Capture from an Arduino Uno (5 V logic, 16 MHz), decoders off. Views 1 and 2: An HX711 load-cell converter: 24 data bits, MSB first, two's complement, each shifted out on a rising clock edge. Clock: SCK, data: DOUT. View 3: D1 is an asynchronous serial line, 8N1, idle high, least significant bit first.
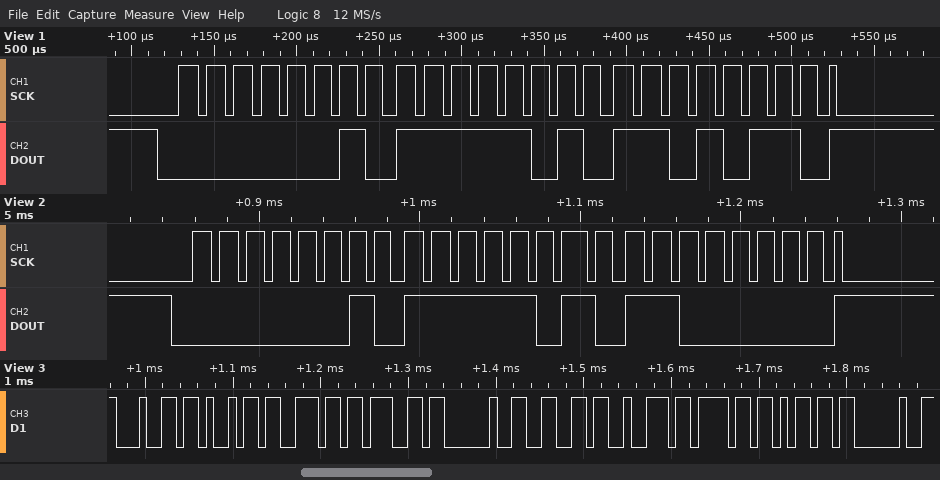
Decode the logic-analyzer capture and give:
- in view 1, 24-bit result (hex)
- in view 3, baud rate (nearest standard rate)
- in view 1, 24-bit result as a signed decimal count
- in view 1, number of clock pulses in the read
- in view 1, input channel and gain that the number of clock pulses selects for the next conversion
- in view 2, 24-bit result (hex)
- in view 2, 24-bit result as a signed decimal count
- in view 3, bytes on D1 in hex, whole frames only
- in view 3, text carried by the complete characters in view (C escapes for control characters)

0x02FAD6
115200 baud
195286
25
channel A, gain 128
0x02FAC0
195264
64 69 6E 67 20 66 72 6F 6D 20
"ding from "
